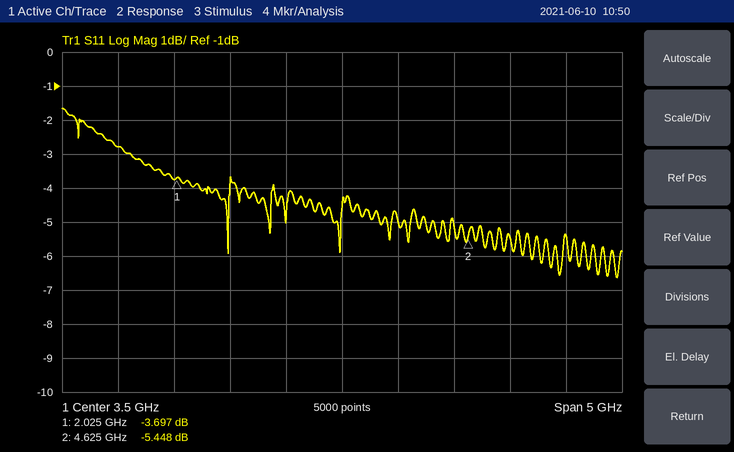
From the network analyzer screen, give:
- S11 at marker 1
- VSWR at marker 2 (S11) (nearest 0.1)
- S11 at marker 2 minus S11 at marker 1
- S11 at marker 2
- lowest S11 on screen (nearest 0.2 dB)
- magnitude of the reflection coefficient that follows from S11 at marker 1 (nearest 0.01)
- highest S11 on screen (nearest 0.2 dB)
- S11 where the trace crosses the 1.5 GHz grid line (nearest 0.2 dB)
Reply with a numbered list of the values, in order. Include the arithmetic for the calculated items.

1. -3.697 dB
2. (1 + 0.5341)/(1 − 0.5341) ≈ 3.3
3. -5.448 − (-3.697) = -1.751 dB
4. -5.448 dB
5. -6.6 dB
6. 10^(-3.697/20) ≈ 0.65
7. -1.6 dB
8. -2.8 dB
